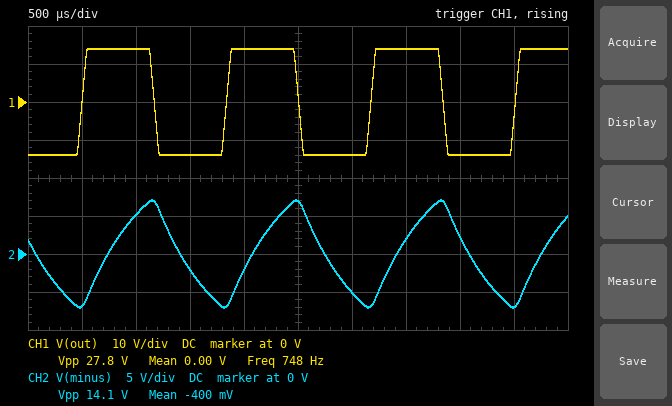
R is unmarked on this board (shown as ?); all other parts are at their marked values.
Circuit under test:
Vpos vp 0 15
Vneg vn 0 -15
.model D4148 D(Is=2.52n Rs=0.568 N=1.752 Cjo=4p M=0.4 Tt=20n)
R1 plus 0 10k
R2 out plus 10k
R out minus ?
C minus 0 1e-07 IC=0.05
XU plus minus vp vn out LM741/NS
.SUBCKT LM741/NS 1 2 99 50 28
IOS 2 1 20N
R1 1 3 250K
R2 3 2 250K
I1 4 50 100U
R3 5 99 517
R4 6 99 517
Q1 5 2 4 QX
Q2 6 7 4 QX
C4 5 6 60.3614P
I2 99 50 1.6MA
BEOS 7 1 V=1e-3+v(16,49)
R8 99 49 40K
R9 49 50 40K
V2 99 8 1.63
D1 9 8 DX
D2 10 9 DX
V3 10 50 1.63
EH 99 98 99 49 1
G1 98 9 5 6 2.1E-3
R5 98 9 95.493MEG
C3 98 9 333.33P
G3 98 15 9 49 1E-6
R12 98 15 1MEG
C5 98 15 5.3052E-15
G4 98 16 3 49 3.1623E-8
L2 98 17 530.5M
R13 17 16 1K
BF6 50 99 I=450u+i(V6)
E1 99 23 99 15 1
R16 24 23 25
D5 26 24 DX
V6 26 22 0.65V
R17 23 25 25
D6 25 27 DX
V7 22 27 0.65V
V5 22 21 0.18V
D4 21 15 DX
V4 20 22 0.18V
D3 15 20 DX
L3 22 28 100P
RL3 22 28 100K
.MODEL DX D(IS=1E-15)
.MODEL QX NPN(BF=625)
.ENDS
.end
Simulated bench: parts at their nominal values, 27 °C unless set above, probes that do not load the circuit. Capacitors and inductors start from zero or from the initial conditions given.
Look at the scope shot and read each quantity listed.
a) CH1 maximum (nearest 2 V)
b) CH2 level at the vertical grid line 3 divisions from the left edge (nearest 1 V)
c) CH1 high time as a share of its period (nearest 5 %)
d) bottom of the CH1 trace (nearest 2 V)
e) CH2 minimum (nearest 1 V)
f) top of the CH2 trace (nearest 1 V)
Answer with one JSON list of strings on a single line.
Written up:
["14 V", "-2 V", "50 %", "-14 V", "-7 V", "7 V"]
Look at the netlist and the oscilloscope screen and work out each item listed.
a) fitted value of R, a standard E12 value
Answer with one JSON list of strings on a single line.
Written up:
["5.6 kΩ"]
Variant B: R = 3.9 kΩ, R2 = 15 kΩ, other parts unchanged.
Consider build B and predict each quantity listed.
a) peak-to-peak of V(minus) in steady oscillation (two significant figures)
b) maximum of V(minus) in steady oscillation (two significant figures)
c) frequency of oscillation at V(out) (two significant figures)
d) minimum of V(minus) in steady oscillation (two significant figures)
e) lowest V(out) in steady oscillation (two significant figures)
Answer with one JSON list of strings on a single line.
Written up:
["12 V", "5.8 V", "1.3 kHz", "-5.8 V", "-14 V"]
